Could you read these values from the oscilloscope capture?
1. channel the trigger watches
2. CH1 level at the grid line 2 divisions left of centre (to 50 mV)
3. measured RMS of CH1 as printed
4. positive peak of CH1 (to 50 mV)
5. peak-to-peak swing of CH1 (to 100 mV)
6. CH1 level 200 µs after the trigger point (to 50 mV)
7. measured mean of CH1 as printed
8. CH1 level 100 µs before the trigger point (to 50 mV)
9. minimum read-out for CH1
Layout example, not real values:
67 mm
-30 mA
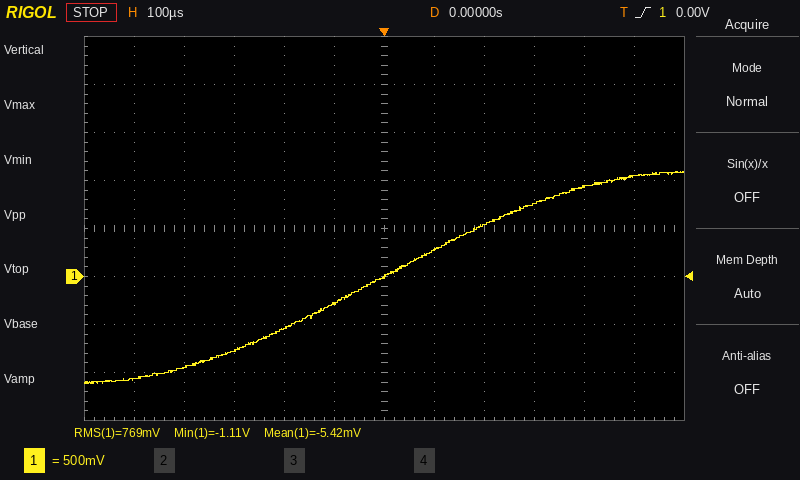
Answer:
CH1
-550 mV
769 mV
1.10 V
2.20 V
550 mV
-5.42 mV
-300 mV
-1.11 V
